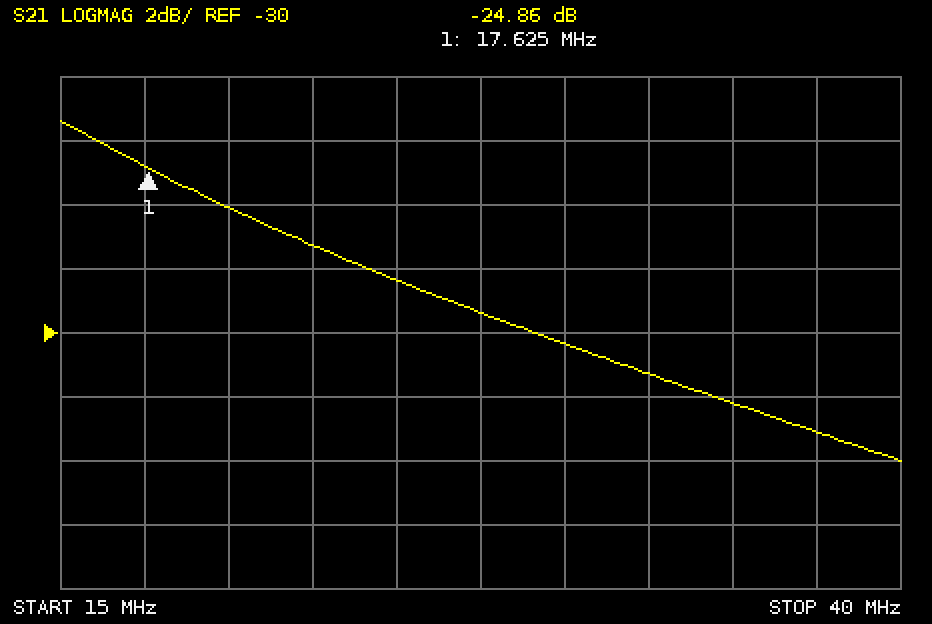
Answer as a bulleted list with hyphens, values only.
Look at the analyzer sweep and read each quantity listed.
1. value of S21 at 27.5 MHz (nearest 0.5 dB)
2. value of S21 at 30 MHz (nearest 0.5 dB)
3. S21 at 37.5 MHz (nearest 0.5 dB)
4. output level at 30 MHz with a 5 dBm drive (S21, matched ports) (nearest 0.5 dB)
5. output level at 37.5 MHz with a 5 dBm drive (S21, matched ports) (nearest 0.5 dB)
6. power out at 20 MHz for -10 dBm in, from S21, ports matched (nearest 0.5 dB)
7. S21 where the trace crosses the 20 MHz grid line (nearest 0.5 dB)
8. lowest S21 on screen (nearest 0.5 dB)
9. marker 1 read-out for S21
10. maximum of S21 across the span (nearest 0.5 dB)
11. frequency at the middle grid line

- -29.5 dB
- -30.5 dB
- -33.0 dB
- -25.5 dBm
- -28.0 dBm
- -36.0 dBm
- -26.0 dB
- -34.0 dB
- -24.86 dB
- -23.5 dB
- 27.5 MHz
